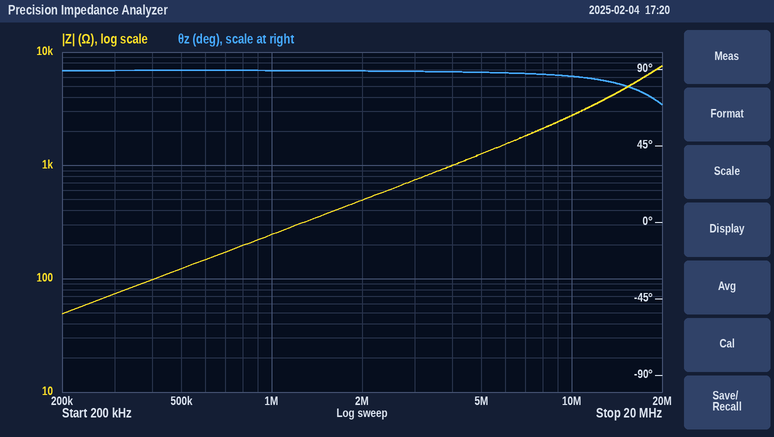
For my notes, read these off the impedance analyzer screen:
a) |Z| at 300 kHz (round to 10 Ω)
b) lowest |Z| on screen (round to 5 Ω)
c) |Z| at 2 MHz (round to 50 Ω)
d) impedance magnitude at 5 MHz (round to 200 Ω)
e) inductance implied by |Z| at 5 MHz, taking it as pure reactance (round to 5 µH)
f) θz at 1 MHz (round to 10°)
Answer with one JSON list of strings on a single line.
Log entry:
["70 Ω", "50 Ω", "500 Ω", "1.2 kΩ", "40 µH", "90°"]
